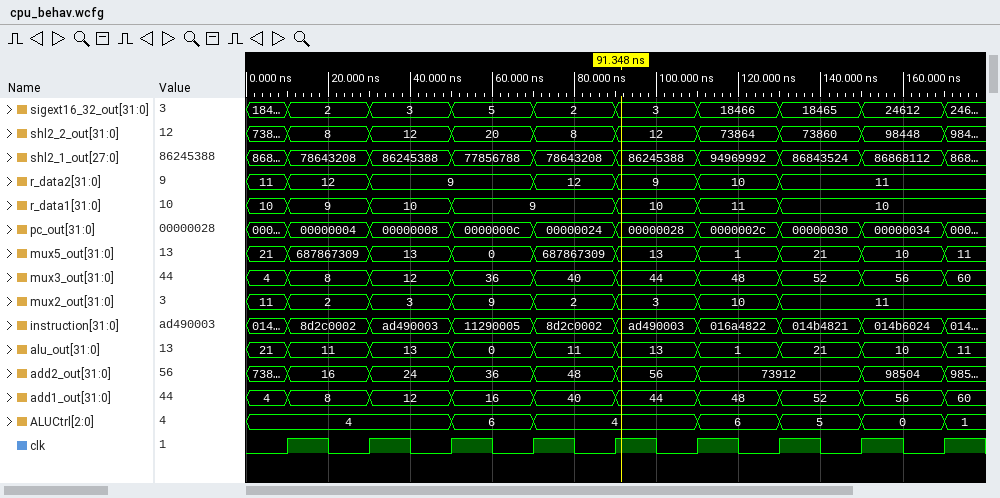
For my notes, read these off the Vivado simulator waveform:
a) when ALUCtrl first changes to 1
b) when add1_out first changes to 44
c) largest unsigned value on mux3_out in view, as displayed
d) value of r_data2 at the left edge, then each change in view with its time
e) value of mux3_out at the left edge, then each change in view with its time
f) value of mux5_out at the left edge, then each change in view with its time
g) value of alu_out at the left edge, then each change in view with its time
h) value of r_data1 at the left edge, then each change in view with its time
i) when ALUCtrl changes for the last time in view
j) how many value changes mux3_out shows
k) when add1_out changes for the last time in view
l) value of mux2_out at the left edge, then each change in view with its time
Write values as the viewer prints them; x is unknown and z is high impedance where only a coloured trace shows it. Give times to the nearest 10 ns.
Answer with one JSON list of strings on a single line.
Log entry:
["170 ns", "90 ns", "60", "11, 12 at 10 ns, 9 at 30 ns, 12 at 70 ns, 9 at 90 ns, 10 at 110 ns, 11 at 130 ns", "4, 8 at 10 ns, 12 at 30 ns, 36 at 50 ns, 40 at 70 ns, 44 at 90 ns, 48 at 110 ns, 52 at 130 ns, 56 at 150 ns, 60 at 170 ns", "21, 687867309 at 10 ns, 13 at 30 ns, 0 at 50 ns, 687867309 at 70 ns, 13 at 90 ns, 1 at 110 ns, 21 at 130 ns, 10 at 150 ns, 11 at 170 ns", "21, 11 at 10 ns, 13 at 30 ns, 0 at 50 ns, 11 at 70 ns, 13 at 90 ns, 1 at 110 ns, 21 at 130 ns, 10 at 150 ns, 11 at 170 ns", "10, 9 at 10 ns, 10 at 30 ns, 9 at 50 ns, 10 at 90 ns, 11 at 110 ns, 10 at 130 ns", "170 ns", "9", "170 ns", "11, 2 at 10 ns, 3 at 30 ns, 9 at 50 ns, 2 at 70 ns, 3 at 90 ns, 10 at 110 ns, 11 at 130 ns"]
